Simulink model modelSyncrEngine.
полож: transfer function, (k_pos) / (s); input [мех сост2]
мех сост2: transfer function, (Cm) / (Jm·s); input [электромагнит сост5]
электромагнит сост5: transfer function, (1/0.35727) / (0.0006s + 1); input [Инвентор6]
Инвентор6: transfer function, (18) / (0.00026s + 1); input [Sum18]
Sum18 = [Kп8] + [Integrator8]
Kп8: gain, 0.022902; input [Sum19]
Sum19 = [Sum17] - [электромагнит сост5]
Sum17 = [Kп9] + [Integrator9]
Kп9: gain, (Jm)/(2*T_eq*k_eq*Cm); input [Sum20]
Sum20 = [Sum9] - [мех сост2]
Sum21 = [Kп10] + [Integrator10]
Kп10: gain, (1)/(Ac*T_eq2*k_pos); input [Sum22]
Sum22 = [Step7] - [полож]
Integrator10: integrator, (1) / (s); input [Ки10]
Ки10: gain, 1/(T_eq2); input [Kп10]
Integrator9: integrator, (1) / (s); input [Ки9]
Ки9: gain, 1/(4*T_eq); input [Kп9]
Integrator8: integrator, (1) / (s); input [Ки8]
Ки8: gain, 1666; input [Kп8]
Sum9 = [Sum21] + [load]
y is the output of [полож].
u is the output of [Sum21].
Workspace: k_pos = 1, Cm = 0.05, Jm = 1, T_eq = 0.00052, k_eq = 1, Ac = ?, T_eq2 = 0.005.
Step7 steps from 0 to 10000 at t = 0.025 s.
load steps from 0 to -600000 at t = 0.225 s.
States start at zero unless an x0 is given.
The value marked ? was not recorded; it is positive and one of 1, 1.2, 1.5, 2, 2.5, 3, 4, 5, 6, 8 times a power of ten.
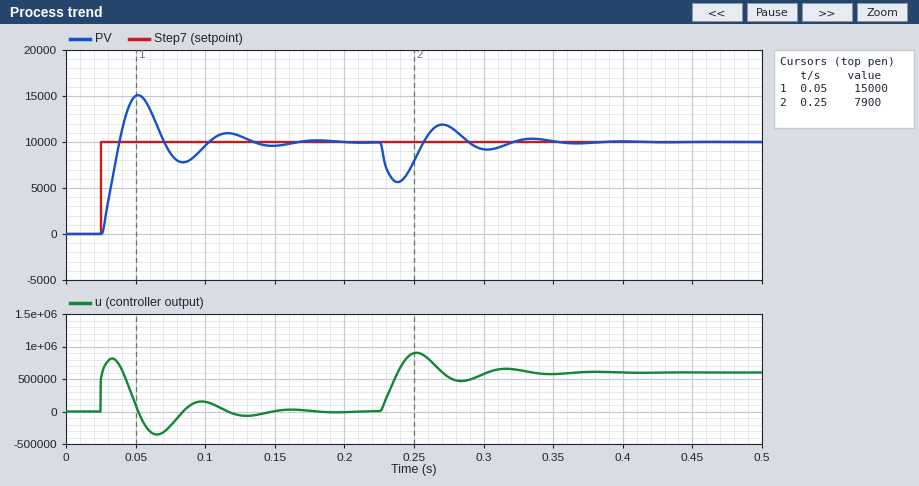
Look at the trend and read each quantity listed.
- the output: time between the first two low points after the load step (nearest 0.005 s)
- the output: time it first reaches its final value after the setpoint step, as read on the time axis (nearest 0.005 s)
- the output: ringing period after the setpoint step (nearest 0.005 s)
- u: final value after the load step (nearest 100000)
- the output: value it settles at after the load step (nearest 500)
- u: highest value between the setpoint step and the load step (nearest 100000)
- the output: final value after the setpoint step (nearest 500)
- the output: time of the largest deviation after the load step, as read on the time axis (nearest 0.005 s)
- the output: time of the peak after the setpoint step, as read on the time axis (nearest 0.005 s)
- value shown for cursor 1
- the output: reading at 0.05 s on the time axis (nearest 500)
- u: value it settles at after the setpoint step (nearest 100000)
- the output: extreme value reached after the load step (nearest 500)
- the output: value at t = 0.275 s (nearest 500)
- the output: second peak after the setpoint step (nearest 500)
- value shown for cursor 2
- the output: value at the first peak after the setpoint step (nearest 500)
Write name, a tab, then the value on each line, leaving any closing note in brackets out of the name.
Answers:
the output: time between the first two low points after the load step	0.065 s
the output: time it first reaches its final value after the setpoint step, as read on the time axis	0.040 s
the output: ringing period after the setpoint step	0.065 s
u: final value after the load step	600000
the output: value it settles at after the load step	10000
u: highest value between the setpoint step and the load step	800000
the output: final value after the setpoint step	10000
the output: time of the largest deviation after the load step, as read on the time axis	0.240 s
the output: time of the peak after the setpoint step, as read on the time axis	0.050 s
value shown for cursor 1	15000
the output: reading at 0.05 s on the time axis	15000
u: value it settles at after the setpoint step	0
the output: extreme value reached after the load step	5500
the output: value at t = 0.275 s	11500
the output: second peak after the setpoint step	11000
value shown for cursor 2	7900
the output: value at the first peak after the setpoint step	15000
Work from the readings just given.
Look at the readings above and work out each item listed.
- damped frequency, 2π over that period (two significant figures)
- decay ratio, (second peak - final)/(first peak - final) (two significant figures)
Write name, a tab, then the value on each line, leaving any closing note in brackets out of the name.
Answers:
damped frequency, 2π over that period	97 rad/s
decay ratio, (second peak - final)/(first peak - final)	0.20
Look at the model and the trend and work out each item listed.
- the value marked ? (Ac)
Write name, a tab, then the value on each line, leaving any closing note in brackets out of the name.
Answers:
the value marked ?	4
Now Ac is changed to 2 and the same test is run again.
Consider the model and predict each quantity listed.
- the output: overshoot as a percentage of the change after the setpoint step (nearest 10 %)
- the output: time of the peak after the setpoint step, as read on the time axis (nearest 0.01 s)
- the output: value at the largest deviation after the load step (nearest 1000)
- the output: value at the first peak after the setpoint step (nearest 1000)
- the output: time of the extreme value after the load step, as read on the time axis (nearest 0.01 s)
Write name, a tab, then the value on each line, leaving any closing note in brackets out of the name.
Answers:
the output: overshoot as a percentage of the change after the setpoint step	40 %
the output: time of the peak after the setpoint step, as read on the time axis	0.04 s
the output: value at the largest deviation after the load step	7000
the output: value at the first peak after the setpoint step	14000
the output: time of the extreme value after the load step, as read on the time axis	0.23 s
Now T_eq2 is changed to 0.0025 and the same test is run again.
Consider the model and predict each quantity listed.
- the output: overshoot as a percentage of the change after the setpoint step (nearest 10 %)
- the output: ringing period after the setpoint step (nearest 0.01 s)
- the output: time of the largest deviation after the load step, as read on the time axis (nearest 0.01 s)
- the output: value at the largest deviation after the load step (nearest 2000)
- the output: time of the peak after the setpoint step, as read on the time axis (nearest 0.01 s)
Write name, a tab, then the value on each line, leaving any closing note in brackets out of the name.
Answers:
the output: overshoot as a percentage of the change after the setpoint step	50 %
the output: ringing period after the setpoint step	0.03 s
the output: time of the largest deviation after the load step, as read on the time axis	0.23 s
the output: value at the largest deviation after the load step	8000
the output: time of the peak after the setpoint step, as read on the time axis	0.04 s
